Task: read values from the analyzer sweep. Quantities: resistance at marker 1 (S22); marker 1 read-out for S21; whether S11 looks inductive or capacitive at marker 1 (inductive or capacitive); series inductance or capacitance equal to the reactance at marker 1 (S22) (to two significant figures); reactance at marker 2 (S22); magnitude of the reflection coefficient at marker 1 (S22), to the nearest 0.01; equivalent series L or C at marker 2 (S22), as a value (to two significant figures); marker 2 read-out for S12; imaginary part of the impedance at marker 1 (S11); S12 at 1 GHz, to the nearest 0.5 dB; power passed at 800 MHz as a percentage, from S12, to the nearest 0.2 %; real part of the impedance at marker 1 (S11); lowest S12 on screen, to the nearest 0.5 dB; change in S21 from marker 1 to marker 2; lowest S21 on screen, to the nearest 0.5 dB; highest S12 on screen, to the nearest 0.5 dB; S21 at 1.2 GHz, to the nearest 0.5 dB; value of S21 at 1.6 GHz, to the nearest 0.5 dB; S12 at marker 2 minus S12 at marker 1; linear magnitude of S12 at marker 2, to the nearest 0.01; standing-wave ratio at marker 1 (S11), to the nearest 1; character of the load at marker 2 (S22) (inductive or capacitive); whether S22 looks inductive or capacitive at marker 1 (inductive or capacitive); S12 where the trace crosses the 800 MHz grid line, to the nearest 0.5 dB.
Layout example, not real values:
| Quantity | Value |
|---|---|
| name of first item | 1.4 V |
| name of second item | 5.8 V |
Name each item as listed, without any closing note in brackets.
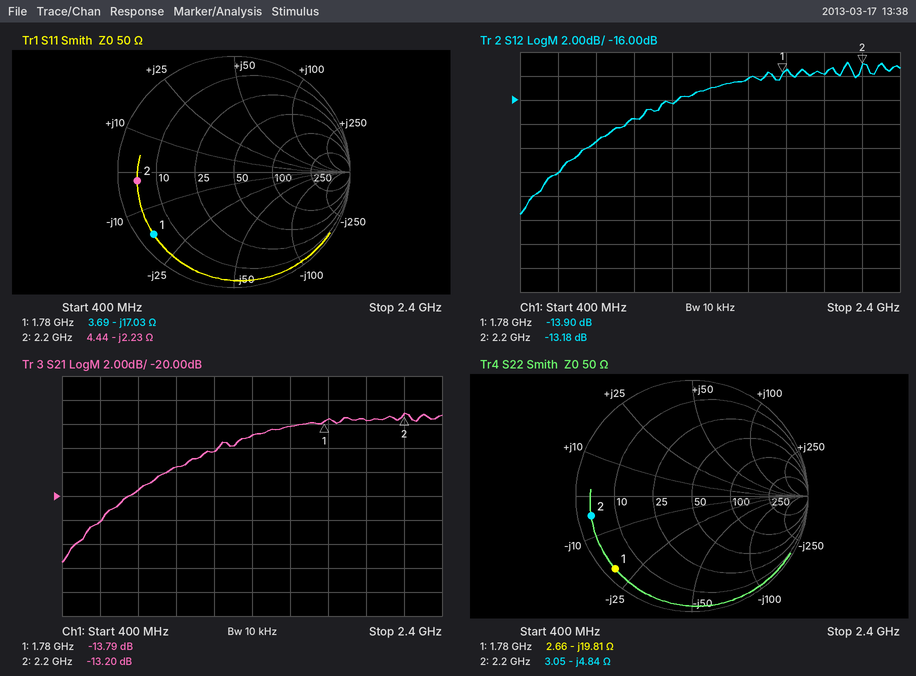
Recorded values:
| Quantity | Value |
|---|---|
| resistance at marker 1 | 2.66 Ω |
| marker 1 read-out for S21 | -13.79 dB |
| whether S11 looks inductive or capacitive at marker 1 | capacitive |
| series inductance or capacitance equal to the reactance at marker 1 (S22) | 4.5 pF |
| reactance at marker 2 | -4.84 Ω |
| magnitude of the reflection coefficient at marker 1 (S22), to the nearest 0.01 | 0.91 |
| equivalent series L or C at marker 2 (S22), as a value | 15 pF |
| marker 2 read-out for S12 | -13.18 dB |
| imaginary part of the impedance at marker 1 | -17.03 Ω |
| S12 at 1 GHz, to the nearest 0.5 dB | -17.5 dB |
| power passed at 800 MHz as a percentage, from S12, to the nearest 0.2 % | 1.2 % |
| real part of the impedance at marker 1 | 3.69 Ω |
| lowest S12 on screen, to the nearest 0.5 dB | -25.5 dB |
| change in S21 from marker 1 to marker 2 | 0.59 dB |
| lowest S21 on screen, to the nearest 0.5 dB | -25.5 dB |
| highest S12 on screen, to the nearest 0.5 dB | -13.0 dB |
| S21 at 1.2 GHz, to the nearest 0.5 dB | -16.5 dB |
| value of S21 at 1.6 GHz, to the nearest 0.5 dB | -14.0 dB |
| S12 at marker 2 minus S12 at marker 1 | 0.72 dB |
| linear magnitude of S12 at marker 2, to the nearest 0.01 | 0.22 |
| standing-wave ratio at marker 1 (S11), to the nearest 1 | 15 |
| character of the load at marker 2 (S22) | capacitive |
| whether S22 looks inductive or capacitive at marker 1 | capacitive |
| S12 where the trace crosses the 800 MHz grid line, to the nearest 0.5 dB | -19.5 dB |
